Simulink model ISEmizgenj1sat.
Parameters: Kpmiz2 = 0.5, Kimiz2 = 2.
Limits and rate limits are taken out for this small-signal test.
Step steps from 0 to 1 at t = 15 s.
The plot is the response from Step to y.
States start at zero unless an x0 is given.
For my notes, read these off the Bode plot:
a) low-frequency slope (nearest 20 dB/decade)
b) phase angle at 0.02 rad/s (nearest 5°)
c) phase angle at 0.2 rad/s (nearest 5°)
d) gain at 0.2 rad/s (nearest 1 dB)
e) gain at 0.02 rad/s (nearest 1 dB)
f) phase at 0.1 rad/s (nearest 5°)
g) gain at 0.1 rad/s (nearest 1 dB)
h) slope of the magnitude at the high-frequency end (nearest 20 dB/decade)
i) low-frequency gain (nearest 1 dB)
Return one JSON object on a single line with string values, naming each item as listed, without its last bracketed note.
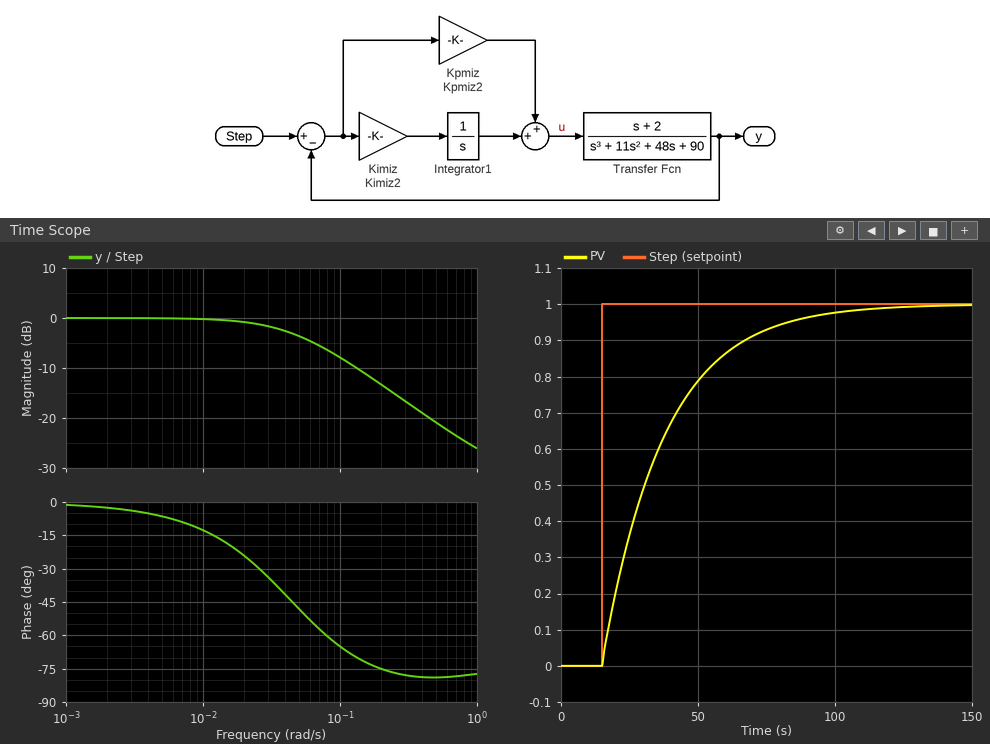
{"low-frequency slope": "0 dB/decade", "phase angle at 0.02 rad/s": "-25°", "phase angle at 0.2 rad/s": "-75°", "gain at 0.2 rad/s": "-13 dB", "gain at 0.02 rad/s": "-1 dB", "phase at 0.1 rad/s": "-65°", "gain at 0.1 rad/s": "-8 dB", "slope of the magnitude at the high-frequency end": "-20 dB/decade", "low-frequency gain": "0 dB"}
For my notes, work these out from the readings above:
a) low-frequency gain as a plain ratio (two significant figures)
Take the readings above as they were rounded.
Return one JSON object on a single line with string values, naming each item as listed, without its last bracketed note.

{"low-frequency gain as a plain ratio": "1.0"}
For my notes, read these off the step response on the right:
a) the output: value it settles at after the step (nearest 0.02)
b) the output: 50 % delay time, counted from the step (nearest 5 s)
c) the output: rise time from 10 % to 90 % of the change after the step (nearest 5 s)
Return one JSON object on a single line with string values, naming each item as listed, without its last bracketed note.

{"the output: value it settles at after the step": "1.00", "the output: 50 % delay time, counted from the step": "15 s", "the output: rise time from 10 % to 90 % of the change after the step": "50 s"}
